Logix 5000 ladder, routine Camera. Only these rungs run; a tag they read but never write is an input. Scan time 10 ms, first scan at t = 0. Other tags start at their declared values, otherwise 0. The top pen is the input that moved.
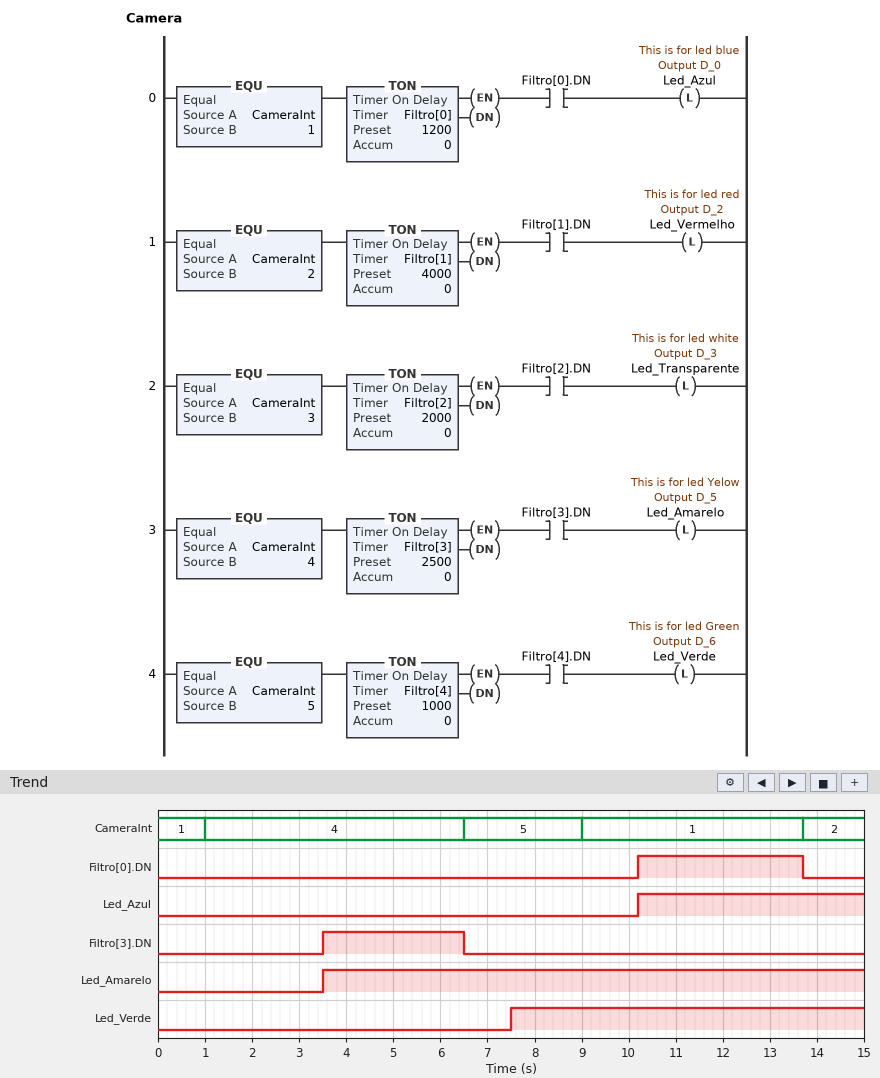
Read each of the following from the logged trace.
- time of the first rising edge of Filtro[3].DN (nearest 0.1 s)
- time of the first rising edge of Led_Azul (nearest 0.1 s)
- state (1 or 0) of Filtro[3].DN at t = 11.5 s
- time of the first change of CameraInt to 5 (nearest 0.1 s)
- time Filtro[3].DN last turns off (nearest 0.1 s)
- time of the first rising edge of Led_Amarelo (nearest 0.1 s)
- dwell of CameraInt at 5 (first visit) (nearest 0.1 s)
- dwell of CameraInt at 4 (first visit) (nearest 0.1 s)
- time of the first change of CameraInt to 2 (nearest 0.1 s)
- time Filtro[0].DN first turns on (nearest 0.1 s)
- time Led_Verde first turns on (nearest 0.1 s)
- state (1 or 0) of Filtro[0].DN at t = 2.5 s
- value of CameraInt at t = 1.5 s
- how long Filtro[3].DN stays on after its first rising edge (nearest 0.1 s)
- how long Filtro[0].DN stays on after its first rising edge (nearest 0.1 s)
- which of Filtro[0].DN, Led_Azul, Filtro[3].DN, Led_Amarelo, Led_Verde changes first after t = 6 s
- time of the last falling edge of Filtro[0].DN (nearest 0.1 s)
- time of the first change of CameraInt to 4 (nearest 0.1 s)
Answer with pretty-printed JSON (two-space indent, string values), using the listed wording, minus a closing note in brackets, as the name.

{
  "time of the first rising edge of Filtro[3].DN": "3.5 s",
  "time of the first rising edge of Led_Azul": "10.2 s",
  "state (1 or 0) of Filtro[3].DN at t = 11.5 s": "0",
  "time of the first change of CameraInt to 5": "6.5 s",
  "time Filtro[3].DN last turns off": "6.5 s",
  "time of the first rising edge of Led_Amarelo": "3.5 s",
  "dwell of CameraInt at 5 (first visit)": "2.5 s",
  "dwell of CameraInt at 4 (first visit)": "5.5 s",
  "time of the first change of CameraInt to 2": "13.7 s",
  "time Filtro[0].DN first turns on": "10.2 s",
  "time Led_Verde first turns on": "7.5 s",
  "state (1 or 0) of Filtro[0].DN at t = 2.5 s": "0",
  "value of CameraInt at t = 1.5 s": "4",
  "how long Filtro[3].DN stays on after its first rising edge": "3.0 s",
  "how long Filtro[0].DN stays on after its first rising edge": "3.5 s",
  "which of Filtro[0].DN, Led_Azul, Filtro[3].DN, Led_Amarelo, Led_Verde changes first after t = 6 s": "Filtro[3].DN",
  "time of the last falling edge of Filtro[0].DN": "13.7 s",
  "time of the first change of CameraInt to 4": "1.0 s"
}
